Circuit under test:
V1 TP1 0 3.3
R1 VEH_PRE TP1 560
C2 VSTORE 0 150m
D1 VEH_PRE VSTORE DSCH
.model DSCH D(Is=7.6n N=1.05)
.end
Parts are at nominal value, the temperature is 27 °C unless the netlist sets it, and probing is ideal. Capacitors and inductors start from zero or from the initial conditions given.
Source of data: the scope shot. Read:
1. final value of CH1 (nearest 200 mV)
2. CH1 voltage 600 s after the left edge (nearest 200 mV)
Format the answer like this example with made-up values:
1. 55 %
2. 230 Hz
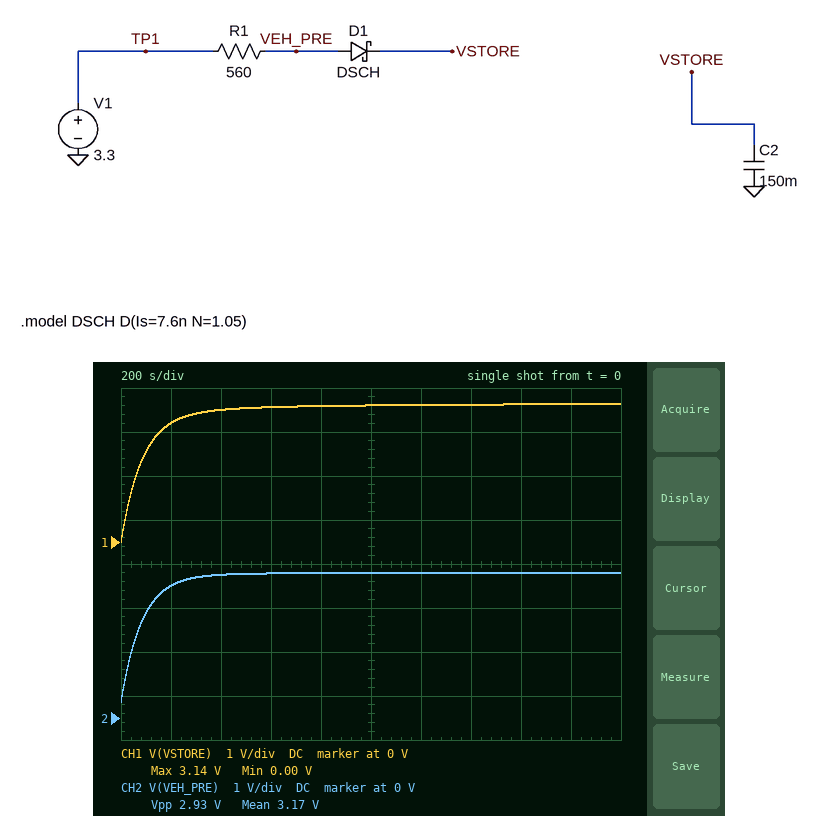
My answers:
1. 3.2 V
2. 3.0 V
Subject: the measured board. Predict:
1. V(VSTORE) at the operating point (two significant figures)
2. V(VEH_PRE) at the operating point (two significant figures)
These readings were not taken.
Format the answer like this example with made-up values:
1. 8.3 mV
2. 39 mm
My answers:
1. 3.3 V
2. 3.3 V
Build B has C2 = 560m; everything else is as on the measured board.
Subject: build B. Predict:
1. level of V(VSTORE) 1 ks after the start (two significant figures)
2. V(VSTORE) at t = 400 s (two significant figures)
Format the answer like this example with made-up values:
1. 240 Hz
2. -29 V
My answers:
1. 2.9 V
2. 2.1 V
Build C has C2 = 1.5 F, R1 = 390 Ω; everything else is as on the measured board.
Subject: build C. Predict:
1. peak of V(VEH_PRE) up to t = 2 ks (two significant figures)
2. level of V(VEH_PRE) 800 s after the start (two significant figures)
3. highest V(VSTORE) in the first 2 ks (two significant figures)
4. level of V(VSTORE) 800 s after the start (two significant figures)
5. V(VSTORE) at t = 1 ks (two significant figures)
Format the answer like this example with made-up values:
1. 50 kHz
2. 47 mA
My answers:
1. 3.2 V
2. 2.5 V
3. 2.9 V
4. 2.2 V
5. 2.4 V
